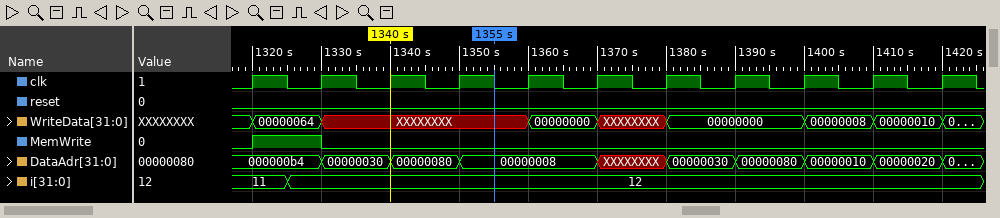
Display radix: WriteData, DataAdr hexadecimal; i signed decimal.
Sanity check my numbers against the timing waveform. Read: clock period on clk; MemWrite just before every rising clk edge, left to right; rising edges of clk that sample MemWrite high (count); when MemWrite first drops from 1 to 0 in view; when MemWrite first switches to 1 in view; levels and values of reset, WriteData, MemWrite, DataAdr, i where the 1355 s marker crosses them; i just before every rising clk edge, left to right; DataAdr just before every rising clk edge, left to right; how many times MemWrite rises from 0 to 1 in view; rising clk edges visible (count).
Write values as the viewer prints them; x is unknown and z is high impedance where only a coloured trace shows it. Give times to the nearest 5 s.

10 s
0 1 0 0 0 0 0 0 0 0 0
1
1330 s
1320 s
reset=0, WriteData=XXXXXXXX, MemWrite=0, DataAdr=00000008, i=12
11, 12, 12, 12, 12, 12, 12, 12, 12, 12, 12
000000b4, 000000b4, 00000030, 00000080, 00000008, 00000008, XXXXXXXX, 00000030, 00000080, 00000010, 00000020
1
11
